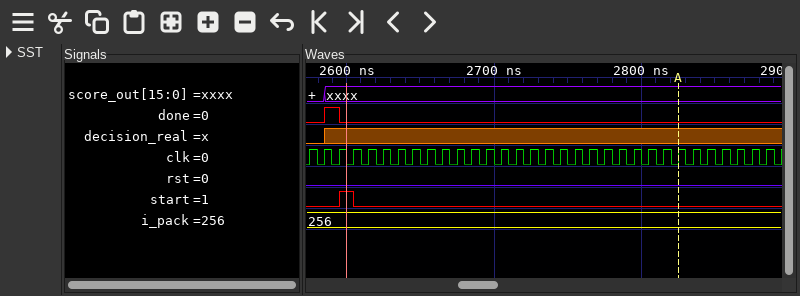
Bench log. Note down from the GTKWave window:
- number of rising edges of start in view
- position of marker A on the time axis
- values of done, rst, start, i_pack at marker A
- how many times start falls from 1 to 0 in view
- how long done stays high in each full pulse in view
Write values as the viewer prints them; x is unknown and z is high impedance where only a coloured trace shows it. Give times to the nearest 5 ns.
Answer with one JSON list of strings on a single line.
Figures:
["1", "2825 ns", "done=0, rst=0, start=0, i_pack=256", "1", "10 ns"]
